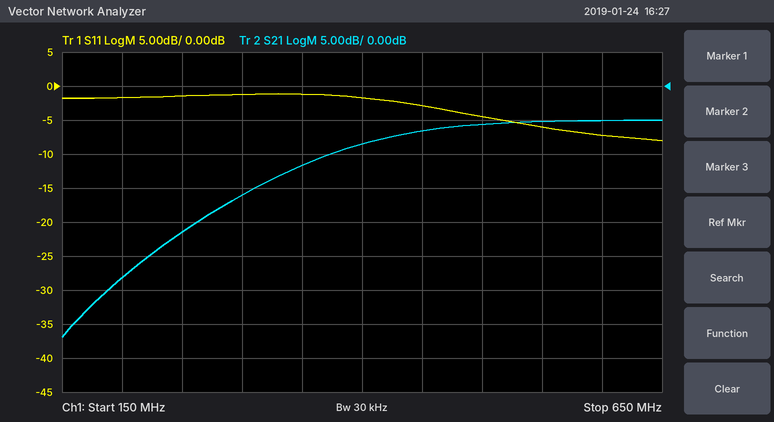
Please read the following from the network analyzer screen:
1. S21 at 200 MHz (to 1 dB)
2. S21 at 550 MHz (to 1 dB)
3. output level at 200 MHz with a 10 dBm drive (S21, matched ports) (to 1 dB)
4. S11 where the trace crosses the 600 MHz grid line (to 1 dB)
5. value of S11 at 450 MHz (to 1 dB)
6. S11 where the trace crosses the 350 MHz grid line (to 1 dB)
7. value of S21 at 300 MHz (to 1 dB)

-28 dB
-5 dB
-18 dBm
-7 dB
-3 dB
-1 dB
-16 dB
